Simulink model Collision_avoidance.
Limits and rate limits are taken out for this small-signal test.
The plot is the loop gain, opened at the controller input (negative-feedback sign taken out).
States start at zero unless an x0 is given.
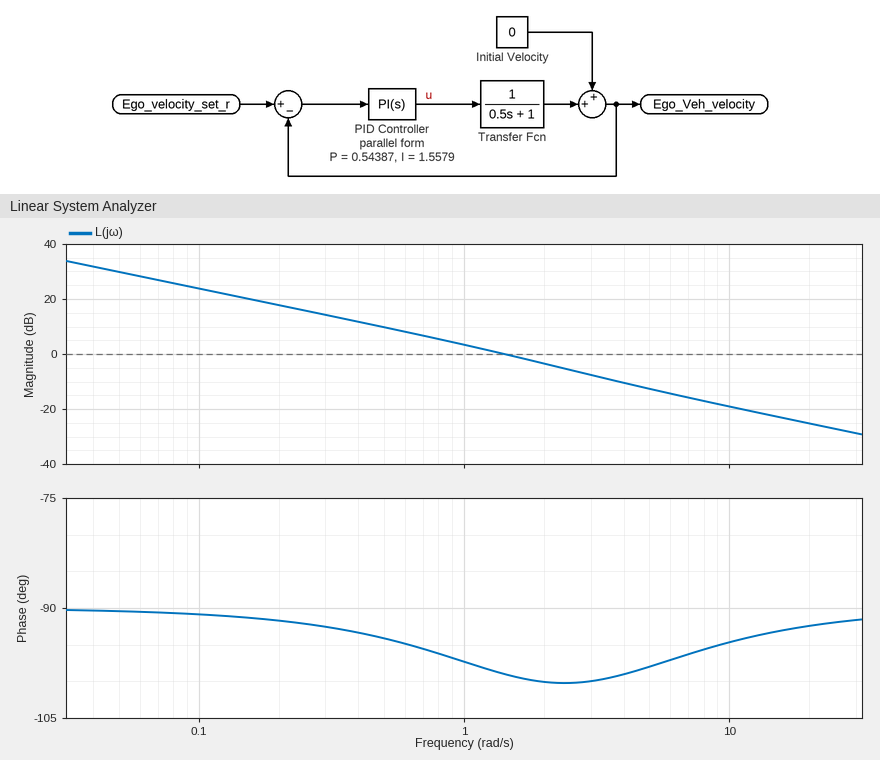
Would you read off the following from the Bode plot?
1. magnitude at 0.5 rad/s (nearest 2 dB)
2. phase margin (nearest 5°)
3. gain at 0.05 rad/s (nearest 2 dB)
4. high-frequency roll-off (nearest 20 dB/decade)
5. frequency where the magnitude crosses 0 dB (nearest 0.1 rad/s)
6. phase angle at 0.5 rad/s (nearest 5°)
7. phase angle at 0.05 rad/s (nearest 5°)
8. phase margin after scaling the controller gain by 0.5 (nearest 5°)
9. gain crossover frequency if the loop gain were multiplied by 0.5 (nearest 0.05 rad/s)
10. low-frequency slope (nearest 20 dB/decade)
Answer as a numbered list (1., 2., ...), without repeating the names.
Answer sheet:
1. 10 dB
2. 80°
3. 30 dB
4. -20 dB/decade
5. 1.4 rad/s
6. -95°
7. -90°
8. 85°
9. 0.75 rad/s
10. -20 dB/decade
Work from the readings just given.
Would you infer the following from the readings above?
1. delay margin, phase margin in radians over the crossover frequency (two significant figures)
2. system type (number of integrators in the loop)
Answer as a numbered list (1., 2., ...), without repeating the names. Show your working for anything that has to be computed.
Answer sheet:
1. 80 × π / 180 / 1.4 = 1.00 s
2. 1
